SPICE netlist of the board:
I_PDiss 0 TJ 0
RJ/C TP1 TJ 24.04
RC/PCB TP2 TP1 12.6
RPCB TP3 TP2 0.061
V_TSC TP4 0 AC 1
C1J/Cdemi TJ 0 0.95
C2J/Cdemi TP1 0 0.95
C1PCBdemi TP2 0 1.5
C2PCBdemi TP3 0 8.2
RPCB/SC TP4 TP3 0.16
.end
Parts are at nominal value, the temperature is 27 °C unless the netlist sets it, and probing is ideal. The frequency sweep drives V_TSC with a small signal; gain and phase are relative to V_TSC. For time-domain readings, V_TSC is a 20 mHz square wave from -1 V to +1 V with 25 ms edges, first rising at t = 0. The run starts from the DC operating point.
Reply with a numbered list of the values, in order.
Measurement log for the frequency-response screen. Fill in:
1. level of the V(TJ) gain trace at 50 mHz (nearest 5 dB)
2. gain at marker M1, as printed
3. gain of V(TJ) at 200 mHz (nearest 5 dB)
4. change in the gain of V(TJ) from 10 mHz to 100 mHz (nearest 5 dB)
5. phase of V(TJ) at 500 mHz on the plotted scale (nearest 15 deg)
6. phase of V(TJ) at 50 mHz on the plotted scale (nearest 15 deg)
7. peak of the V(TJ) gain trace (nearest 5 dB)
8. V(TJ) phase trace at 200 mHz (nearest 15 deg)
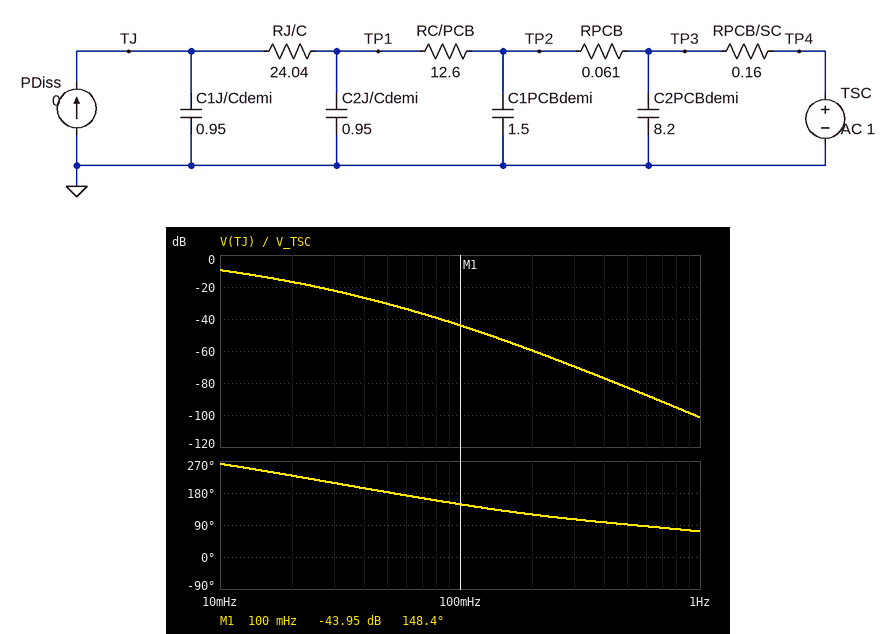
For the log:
1. -30 dB
2. -43.95 dB
3. -60 dB
4. -35 dB
5. 90 deg
6. 180 deg
7. -10 dB
8. 120 deg
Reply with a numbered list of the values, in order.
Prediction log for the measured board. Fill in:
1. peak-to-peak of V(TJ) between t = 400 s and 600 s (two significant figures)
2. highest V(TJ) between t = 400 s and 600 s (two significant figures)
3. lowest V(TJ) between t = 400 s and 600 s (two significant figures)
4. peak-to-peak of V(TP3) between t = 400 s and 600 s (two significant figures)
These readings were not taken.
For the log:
1. 380 mV
2. 190 mV
3. -190 mV
4. 2.0 V
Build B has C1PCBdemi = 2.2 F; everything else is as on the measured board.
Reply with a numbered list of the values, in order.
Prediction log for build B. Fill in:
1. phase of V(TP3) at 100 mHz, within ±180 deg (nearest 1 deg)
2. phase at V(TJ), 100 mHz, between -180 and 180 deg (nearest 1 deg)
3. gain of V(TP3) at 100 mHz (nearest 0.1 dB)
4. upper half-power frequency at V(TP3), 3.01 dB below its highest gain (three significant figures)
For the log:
1. -45 deg
2. 145 deg
3. -3.3 dB
4. 93.0 mHz
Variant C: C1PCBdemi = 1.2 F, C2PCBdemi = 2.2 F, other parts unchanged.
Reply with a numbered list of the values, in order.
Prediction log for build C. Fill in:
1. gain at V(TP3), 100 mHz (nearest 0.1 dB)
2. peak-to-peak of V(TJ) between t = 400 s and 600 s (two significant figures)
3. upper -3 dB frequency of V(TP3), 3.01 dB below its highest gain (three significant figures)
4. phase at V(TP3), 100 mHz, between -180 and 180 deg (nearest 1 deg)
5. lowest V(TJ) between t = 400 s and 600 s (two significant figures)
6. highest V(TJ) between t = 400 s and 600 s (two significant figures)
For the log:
1. -0.6 dB
2. 390 mV
3. 278 mHz
4. -19 deg
5. -200 mV
6. 200 mV
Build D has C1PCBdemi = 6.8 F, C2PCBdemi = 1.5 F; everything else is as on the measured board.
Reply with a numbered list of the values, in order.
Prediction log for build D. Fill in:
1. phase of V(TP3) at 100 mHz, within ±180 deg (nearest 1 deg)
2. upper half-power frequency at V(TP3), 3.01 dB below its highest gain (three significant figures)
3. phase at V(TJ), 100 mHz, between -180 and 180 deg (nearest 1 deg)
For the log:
1. -34 deg
2. 99.7 mHz
3. 147 deg
